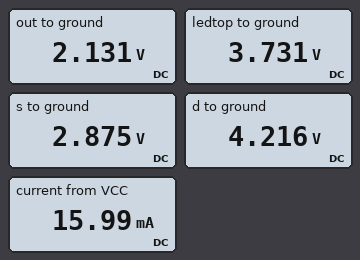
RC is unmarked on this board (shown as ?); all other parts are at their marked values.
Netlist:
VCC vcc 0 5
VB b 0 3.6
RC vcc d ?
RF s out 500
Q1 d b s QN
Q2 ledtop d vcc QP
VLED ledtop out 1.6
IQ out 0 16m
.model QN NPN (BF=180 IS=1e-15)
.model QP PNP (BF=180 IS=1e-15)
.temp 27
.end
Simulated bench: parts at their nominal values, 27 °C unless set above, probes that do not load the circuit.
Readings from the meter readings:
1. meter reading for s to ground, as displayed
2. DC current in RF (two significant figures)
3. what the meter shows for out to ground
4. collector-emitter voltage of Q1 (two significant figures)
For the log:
2.875 V
1.5 mA
2.131 V
1.3 V
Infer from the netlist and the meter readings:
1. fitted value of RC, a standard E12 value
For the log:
560 Ω
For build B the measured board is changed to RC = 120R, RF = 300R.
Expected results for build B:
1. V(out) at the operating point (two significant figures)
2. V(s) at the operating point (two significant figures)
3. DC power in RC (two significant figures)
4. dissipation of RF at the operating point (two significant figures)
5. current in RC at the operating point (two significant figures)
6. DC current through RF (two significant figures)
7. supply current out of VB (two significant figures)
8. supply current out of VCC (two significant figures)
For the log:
880 mV
2.8 V
5.0 mW
13 mW
6.4 mA
6.5 mA
36 µA
16 mA
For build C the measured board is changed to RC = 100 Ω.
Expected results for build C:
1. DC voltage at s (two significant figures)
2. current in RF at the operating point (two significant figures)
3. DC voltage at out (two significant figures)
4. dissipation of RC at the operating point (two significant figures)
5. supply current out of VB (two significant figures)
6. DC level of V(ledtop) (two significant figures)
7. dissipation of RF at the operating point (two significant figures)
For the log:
2.8 V
7.8 mA
-1.1 V
5.9 mW
43 µA
540 mV
30 mW
